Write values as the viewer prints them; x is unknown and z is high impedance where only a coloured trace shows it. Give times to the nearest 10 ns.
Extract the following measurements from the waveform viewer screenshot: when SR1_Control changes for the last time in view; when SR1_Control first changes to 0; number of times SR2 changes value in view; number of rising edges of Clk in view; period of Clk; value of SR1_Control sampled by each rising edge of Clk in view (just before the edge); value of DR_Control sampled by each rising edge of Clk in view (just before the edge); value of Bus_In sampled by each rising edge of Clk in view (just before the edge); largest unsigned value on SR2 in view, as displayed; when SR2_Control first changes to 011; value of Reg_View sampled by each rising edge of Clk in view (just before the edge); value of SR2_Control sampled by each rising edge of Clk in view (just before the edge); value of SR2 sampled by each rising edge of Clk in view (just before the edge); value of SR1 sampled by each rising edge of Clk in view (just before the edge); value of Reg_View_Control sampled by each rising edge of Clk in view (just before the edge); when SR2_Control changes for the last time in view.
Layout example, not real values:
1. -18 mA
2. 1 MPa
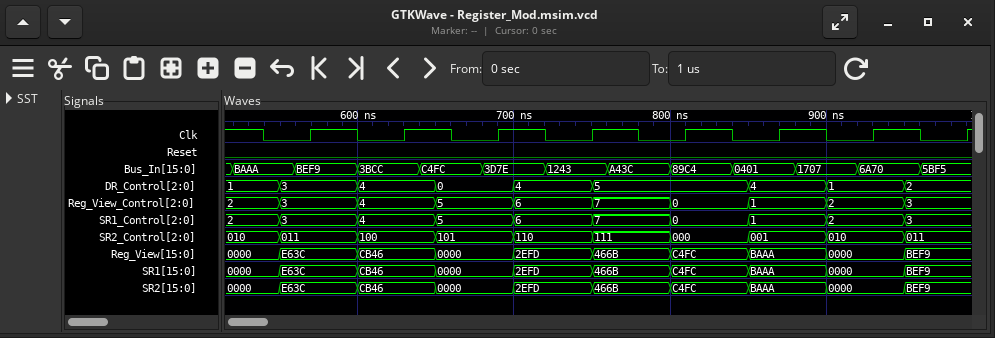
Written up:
1. 950 ns
2. 800 ns
3. 9
4. 8
5. 60 ns
6. 3, 4, 5, 6, 0, 1, 2, 3
7. 3, 4, 0, 4, 5, 4, 1, 2
8. BEF9, 3BCC, 3D7E, 1243, 89C4, 0401, 6A70, 5BF5
9. E63C
10. 550 ns
11. E63C, CB46, 0000, 2EFD, C4FC, BAAA, 0000, BEF9
12. 011, 100, 101, 110, 000, 001, 010, 011
13. E63C, CB46, 0000, 2EFD, C4FC, BAAA, 0000, BEF9
14. E63C, CB46, 0000, 2EFD, C4FC, BAAA, 0000, BEF9
15. 3, 4, 5, 6, 0, 1, 2, 3
16. 950 ns
